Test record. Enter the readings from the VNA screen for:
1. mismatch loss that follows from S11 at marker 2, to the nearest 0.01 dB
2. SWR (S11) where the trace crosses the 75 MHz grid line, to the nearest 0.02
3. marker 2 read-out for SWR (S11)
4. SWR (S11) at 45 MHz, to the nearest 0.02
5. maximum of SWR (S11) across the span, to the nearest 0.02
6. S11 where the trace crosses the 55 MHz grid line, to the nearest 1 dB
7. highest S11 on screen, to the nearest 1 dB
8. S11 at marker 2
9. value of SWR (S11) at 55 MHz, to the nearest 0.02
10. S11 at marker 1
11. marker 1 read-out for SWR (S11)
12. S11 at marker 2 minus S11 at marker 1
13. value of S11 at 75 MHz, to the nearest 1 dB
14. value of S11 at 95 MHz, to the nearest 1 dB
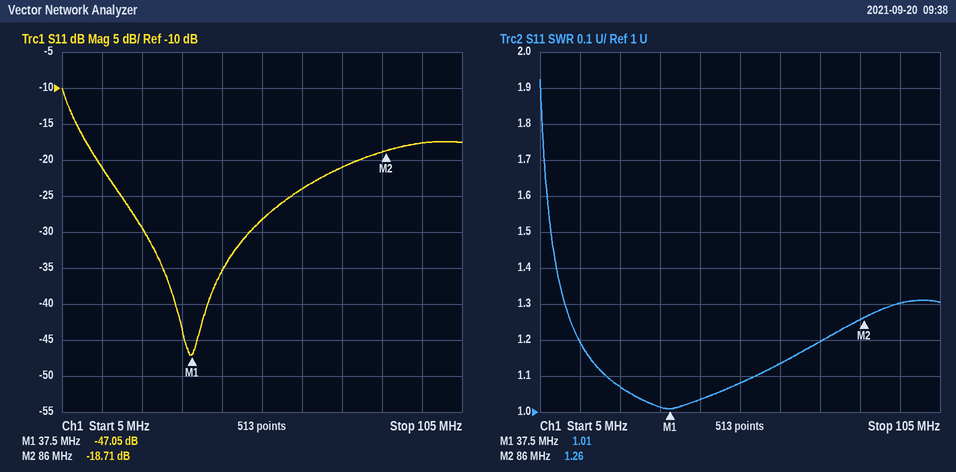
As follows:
0.06 dB
1.20
1.26
1.04
1.92
-28 dB
-10 dB
-18.71 dB
1.08
-47.05 dB
1.01
28.34 dB
-21 dB
-18 dB
